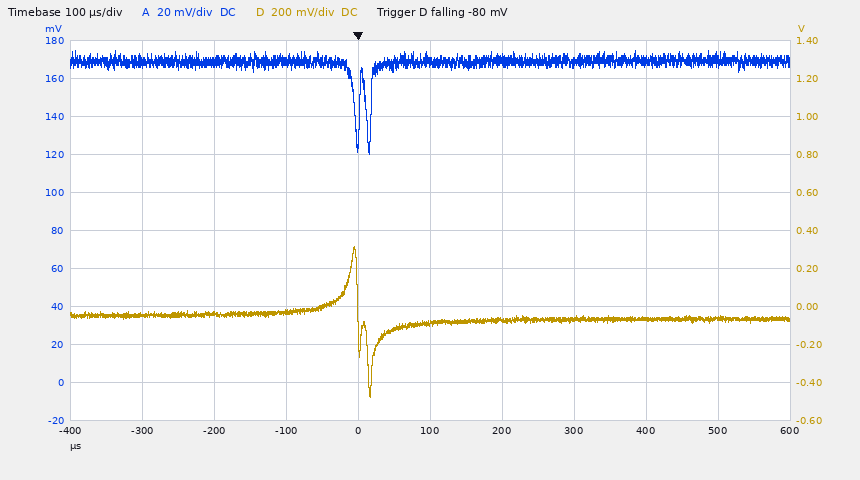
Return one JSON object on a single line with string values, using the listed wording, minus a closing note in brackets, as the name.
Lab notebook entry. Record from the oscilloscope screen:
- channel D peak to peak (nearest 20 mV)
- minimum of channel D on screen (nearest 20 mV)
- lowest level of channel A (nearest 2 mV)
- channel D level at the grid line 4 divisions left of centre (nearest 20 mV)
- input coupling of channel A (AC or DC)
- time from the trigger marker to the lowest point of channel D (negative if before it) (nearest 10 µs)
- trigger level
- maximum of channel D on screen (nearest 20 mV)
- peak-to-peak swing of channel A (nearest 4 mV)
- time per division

{"channel D peak to peak": "800 mV", "minimum of channel D on screen": "-480 mV", "lowest level of channel A": "120 mV", "channel D level at the grid line 4 divisions left of centre": "-40 mV", "input coupling of channel A": "DC", "time from the trigger marker to the lowest point of channel D (negative if before it)": "+20 µs", "trigger level": "-80 mV", "maximum of channel D on screen": "320 mV", "peak-to-peak swing of channel A": "56 mV", "time per division": "100 µs"}
